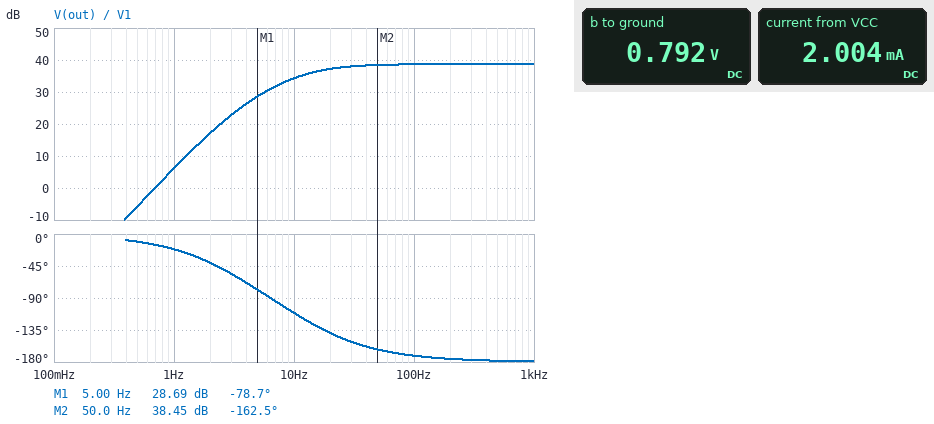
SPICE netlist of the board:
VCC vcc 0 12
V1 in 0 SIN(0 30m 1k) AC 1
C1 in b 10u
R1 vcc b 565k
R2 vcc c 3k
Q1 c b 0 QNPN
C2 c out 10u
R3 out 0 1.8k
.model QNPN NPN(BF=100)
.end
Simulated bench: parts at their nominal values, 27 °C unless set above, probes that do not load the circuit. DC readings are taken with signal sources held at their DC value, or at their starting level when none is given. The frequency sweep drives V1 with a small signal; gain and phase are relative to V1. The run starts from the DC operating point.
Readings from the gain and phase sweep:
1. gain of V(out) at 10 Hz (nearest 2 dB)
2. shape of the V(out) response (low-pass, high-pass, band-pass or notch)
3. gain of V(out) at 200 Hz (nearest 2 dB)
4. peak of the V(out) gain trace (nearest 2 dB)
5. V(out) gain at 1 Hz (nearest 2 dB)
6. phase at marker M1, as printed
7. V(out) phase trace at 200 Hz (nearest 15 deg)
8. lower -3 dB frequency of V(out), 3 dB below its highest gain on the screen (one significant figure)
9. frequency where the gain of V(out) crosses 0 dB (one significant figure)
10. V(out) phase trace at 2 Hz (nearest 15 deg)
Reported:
34 dB
high-pass
38 dB
38 dB
6 dB
-78.7 deg
-180 deg
10 Hz
700 mHz
-45 deg
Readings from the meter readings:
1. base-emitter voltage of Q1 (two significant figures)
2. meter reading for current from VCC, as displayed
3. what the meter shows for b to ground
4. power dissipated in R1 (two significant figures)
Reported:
790 mV
2.004 mA
0.792 V
220 µW
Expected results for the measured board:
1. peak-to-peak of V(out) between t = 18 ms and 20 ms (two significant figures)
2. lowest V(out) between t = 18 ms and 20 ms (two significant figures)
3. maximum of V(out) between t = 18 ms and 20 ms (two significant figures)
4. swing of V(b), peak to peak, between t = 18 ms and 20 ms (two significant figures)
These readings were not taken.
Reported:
5.0 V
-3.2 V
1.8 V
60 mV
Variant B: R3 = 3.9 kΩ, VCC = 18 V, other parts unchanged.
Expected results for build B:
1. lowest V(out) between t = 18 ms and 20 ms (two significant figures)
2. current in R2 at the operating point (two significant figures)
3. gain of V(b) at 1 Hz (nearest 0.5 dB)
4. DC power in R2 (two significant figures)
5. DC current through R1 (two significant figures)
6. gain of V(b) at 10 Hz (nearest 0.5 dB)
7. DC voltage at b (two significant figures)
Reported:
-7.0 V
3.0 mA
-25.5 dB
28 mW
30 µA
-6.5 dB
800 mV
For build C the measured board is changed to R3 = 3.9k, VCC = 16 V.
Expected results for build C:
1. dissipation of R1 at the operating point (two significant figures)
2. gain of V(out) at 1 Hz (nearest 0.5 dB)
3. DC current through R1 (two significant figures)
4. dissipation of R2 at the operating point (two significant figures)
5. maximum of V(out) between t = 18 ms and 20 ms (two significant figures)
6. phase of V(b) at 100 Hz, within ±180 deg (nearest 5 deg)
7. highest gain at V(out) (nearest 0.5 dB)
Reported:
410 µW
12.5 dB
27 µA
22 mW
3.6 V
10 deg
45.0 dB
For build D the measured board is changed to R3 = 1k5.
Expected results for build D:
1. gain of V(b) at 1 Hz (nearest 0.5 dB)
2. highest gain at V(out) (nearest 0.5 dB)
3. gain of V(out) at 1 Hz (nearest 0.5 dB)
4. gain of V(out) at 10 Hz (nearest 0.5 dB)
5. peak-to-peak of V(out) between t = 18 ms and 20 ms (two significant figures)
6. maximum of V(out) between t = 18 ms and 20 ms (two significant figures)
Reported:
-22.0 dB
37.5 dB
4.5 dB
33.0 dB
4.5 V
1.6 V
